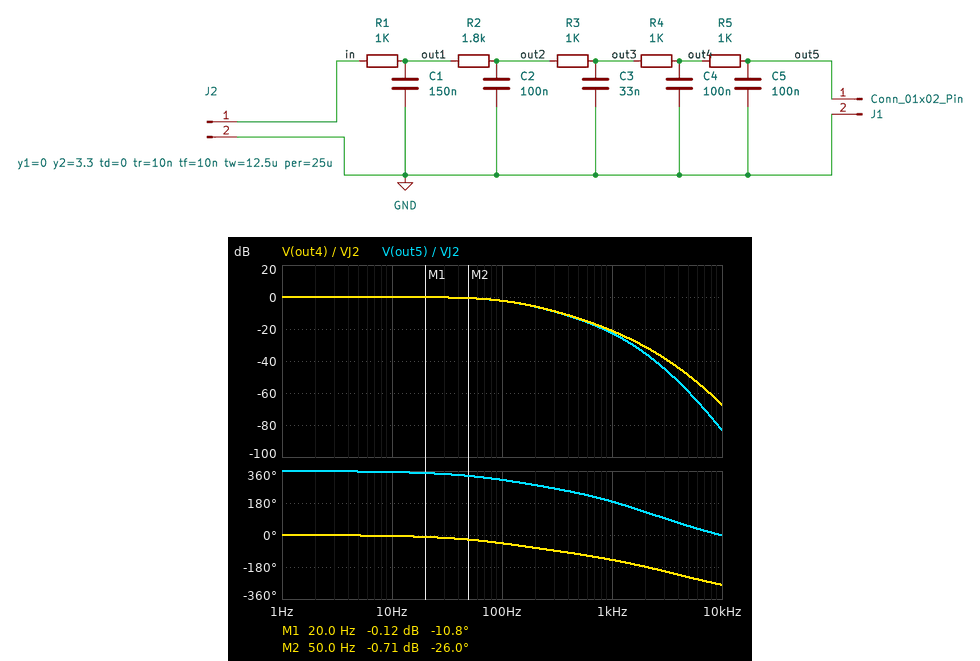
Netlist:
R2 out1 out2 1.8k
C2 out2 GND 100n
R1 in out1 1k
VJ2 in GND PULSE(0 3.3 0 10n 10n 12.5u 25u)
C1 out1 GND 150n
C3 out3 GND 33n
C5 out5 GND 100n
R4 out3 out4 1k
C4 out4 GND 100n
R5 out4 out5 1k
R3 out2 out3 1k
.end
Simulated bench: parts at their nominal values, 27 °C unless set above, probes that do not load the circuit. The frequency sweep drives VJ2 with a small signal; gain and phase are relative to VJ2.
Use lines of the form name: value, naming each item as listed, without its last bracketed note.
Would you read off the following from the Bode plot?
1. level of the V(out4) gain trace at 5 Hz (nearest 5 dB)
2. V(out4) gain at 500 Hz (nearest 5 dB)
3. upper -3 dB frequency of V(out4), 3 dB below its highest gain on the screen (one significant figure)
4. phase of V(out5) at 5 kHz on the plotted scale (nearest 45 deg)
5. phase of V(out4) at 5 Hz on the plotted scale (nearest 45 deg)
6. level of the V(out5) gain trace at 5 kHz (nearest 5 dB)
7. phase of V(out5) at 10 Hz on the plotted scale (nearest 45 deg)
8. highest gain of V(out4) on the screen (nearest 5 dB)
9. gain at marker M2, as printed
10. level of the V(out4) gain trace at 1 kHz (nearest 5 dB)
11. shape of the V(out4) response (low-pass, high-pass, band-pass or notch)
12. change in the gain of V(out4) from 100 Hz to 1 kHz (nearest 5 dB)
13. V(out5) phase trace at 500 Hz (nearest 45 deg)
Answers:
level of the V(out4) gain trace at 5 Hz: 0 dB
V(out4) gain at 500 Hz: -15 dB
upper -3 dB frequency of V(out4), 3 dB below its highest gain on the screen: 100 Hz
phase of V(out5) at 5 kHz on the plotted scale: 45 deg
phase of V(out4) at 5 Hz on the plotted scale: 0 deg
level of the V(out5) gain trace at 5 kHz: -60 dB
phase of V(out5) at 10 Hz on the plotted scale: 360 deg
highest gain of V(out4) on the screen: 0 dB
gain at marker M2, as printed: -0.71 dB
level of the V(out4) gain trace at 1 kHz: -20 dB
shape of the V(out4) response: low-pass
change in the gain of V(out4) from 100 Hz to 1 kHz: -20 dB
V(out5) phase trace at 500 Hz: 225 deg
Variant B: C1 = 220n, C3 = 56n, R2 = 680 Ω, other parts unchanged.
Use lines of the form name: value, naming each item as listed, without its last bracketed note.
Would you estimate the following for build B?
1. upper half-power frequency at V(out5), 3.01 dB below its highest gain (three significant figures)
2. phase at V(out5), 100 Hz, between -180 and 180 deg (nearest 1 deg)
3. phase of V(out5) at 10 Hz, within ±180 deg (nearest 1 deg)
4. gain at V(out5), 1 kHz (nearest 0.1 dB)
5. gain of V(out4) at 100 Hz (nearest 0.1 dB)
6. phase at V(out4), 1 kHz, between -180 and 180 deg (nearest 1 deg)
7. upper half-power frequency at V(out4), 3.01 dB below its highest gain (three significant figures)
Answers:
upper half-power frequency at V(out5), 3.01 dB below its highest gain: 144 Hz
phase at V(out5), 100 Hz, between -180 and 180 deg: -45 deg
phase of V(out5) at 10 Hz, within ±180 deg: -5 deg
gain at V(out5), 1 kHz: -21.3 dB
gain of V(out4) at 100 Hz: -1.7 dB
phase at V(out4), 1 kHz, between -180 and 180 deg: -139 deg
upper half-power frequency at V(out4), 3.01 dB below its highest gain: 145 Hz
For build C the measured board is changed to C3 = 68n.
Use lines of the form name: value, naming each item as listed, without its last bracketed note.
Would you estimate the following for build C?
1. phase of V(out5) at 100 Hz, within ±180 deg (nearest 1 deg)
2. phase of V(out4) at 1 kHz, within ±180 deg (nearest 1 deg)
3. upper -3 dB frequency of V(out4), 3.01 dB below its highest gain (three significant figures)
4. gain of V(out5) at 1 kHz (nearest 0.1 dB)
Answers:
phase of V(out5) at 100 Hz, within ±180 deg: -53 deg
phase of V(out4) at 1 kHz, within ±180 deg: -146 deg
upper -3 dB frequency of V(out4), 3.01 dB below its highest gain: 109 Hz
gain of V(out5) at 1 kHz: -23.6 dB
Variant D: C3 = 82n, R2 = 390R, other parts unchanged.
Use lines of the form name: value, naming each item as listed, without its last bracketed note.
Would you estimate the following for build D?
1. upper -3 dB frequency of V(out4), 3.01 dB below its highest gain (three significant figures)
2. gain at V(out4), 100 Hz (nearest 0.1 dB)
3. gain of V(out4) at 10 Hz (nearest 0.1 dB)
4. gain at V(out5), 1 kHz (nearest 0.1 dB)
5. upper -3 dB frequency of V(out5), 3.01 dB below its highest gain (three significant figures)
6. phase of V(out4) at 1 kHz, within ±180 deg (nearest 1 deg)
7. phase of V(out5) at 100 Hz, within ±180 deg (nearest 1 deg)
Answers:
upper -3 dB frequency of V(out4), 3.01 dB below its highest gain: 156 Hz
gain at V(out4), 100 Hz: -1.5 dB
gain of V(out4) at 10 Hz: 0 dB
gain at V(out5), 1 kHz: -19.8 dB
upper -3 dB frequency of V(out5), 3.01 dB below its highest gain: 155 Hz
phase of V(out4) at 1 kHz, within ±180 deg: -130 deg
phase of V(out5) at 100 Hz, within ±180 deg: -42 deg
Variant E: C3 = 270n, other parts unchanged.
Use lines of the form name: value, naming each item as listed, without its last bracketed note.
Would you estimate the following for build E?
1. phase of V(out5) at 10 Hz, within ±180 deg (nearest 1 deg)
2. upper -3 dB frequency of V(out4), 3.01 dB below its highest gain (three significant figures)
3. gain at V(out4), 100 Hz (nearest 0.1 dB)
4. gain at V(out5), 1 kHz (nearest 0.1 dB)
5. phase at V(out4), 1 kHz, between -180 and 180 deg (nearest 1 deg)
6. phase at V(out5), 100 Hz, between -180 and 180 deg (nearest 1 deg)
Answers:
phase of V(out5) at 10 Hz, within ±180 deg: -9 deg
upper -3 dB frequency of V(out4), 3.01 dB below its highest gain: 73.6 Hz
gain at V(out4), 100 Hz: -4.6 dB
gain at V(out5), 1 kHz: -28.4 dB
phase at V(out4), 1 kHz, between -180 and 180 deg: -166 deg
phase at V(out5), 100 Hz, between -180 and 180 deg: -67 deg
